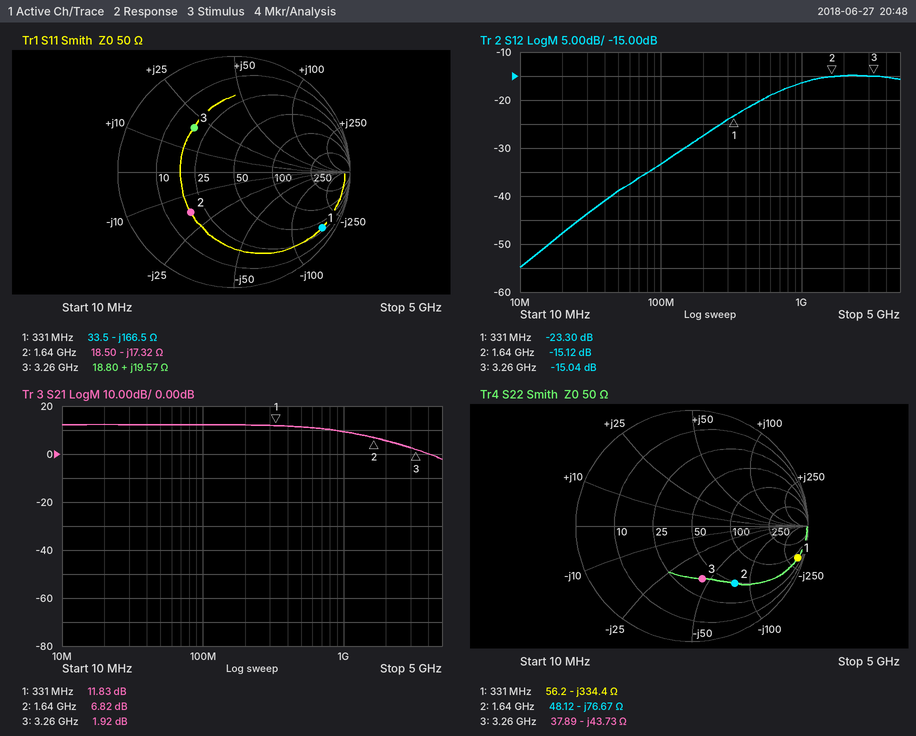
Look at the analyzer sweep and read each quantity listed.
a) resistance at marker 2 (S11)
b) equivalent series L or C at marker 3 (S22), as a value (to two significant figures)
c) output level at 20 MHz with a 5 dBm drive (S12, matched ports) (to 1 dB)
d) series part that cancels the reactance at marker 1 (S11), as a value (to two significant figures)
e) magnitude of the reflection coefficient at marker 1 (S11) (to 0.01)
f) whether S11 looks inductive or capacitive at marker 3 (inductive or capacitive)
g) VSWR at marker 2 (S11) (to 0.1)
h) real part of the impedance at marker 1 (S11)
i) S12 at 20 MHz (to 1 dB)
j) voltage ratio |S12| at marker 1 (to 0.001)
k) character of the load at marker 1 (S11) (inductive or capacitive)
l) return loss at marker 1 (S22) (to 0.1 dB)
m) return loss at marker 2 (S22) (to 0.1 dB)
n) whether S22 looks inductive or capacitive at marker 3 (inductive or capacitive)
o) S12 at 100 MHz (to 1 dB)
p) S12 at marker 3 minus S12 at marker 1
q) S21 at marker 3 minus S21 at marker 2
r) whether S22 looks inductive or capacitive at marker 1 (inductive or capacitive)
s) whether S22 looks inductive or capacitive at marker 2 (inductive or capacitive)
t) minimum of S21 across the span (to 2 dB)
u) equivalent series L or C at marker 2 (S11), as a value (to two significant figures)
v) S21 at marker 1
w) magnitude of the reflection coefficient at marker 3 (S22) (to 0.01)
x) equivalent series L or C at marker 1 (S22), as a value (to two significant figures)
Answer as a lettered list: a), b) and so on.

a) 18.50 Ω
b) 1.1 pF
c) -43 dBm
d) 80 nH
e) 0.90
f) inductive
g) 3.1
h) 33.5 Ω
i) -48 dB
j) 0.068
k) capacitive
l) 0.4 dB
m) 4.2 dB
n) capacitive
o) -33 dB
p) 8.26 dB
q) -4.90 dB
r) capacitive
s) capacitive
t) -2 dB
u) 5.6 pF
v) 11.83 dB
w) 0.46
x) 1.4 pF
